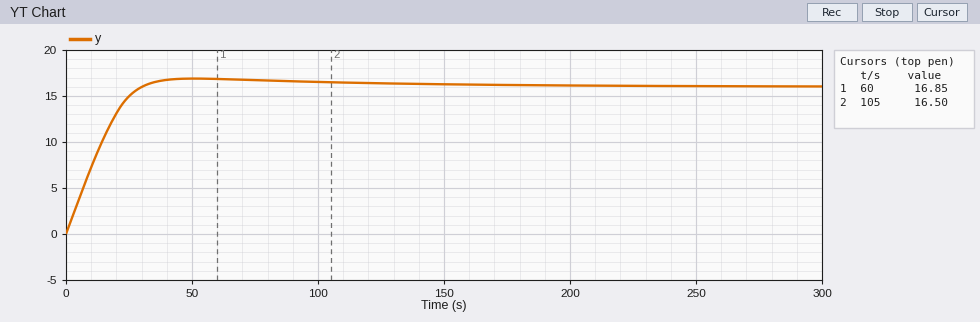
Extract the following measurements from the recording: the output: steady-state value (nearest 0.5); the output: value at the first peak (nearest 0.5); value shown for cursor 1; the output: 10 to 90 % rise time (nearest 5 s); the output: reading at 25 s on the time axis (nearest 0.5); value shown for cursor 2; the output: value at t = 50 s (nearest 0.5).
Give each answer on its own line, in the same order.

16.0
17.0
16.85
20 s
15.0
16.50
17.0
